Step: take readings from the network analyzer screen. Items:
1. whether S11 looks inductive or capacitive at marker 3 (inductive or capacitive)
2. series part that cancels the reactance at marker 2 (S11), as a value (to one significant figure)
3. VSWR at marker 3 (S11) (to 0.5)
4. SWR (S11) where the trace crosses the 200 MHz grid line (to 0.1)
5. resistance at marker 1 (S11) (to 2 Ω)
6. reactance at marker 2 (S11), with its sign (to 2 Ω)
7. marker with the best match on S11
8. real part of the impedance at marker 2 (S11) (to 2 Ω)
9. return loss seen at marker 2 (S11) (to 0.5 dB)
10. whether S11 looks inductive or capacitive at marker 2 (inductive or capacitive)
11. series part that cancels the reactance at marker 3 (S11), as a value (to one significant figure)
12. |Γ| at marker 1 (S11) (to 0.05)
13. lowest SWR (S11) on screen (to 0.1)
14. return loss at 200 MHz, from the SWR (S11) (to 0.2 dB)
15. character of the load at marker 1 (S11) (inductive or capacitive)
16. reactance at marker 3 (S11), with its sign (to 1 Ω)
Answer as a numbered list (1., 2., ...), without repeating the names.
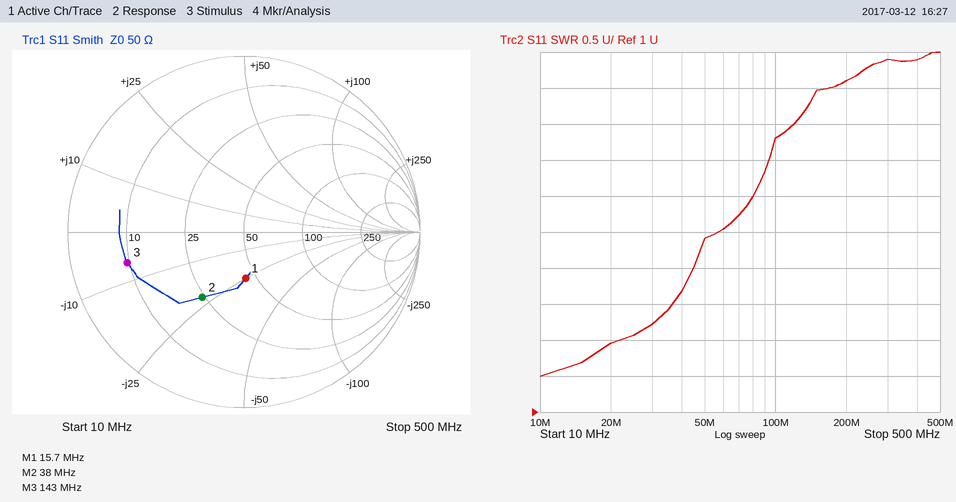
1. capacitive
2. 90 nH
3. 5.5
4. 5.6
5. 44 Ω
6. -22 Ω
7. marker 1
8. 24 Ω
9. 7.0 dB
10. capacitive
11. 7 nH
12. 0.25
13. 1.5
14. 3.2 dB
15. capacitive
16. -6 Ω
